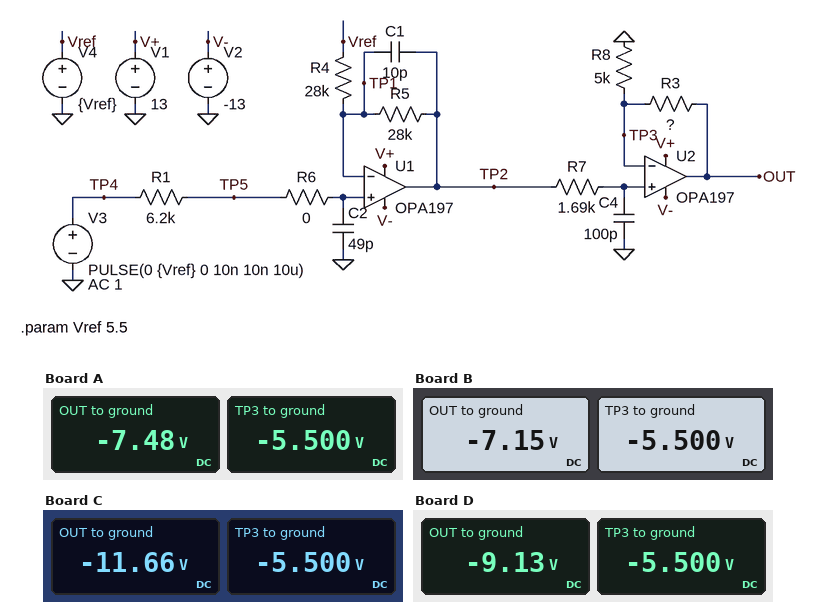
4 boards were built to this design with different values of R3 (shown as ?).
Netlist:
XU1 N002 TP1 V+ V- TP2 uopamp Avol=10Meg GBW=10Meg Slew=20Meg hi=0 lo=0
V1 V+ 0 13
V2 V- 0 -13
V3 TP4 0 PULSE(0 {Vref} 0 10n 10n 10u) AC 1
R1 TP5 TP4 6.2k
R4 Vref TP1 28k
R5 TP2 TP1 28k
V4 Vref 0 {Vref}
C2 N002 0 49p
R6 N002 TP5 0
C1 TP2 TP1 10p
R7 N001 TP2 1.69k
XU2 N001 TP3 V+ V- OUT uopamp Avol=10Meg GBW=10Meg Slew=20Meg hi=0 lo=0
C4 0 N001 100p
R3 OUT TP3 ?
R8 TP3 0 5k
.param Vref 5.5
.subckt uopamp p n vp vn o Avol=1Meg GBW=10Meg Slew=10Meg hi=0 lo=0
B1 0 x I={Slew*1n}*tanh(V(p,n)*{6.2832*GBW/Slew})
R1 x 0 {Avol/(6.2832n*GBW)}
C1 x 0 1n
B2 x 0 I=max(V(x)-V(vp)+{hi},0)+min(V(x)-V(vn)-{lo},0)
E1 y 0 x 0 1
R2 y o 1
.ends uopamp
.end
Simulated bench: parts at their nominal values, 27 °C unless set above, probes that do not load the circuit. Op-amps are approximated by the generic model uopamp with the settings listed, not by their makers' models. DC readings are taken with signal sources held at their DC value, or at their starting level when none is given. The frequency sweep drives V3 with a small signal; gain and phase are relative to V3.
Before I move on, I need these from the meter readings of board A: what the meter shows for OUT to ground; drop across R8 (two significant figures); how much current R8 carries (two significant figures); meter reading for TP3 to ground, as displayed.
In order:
-7.48 V
5.5 V
1.1 mA
-5.500 V
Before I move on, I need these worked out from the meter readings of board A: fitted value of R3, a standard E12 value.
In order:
1.8 kΩ
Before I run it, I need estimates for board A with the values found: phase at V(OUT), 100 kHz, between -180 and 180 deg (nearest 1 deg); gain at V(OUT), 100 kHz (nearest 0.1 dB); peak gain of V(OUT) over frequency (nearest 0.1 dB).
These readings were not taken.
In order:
-20 deg
4.9 dB
5.1 dB
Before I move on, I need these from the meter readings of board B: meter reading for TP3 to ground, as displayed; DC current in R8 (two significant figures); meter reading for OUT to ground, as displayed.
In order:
-5.500 V
1.1 mA
-7.15 V
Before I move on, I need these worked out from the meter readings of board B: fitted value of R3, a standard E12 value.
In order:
1.5 kΩ
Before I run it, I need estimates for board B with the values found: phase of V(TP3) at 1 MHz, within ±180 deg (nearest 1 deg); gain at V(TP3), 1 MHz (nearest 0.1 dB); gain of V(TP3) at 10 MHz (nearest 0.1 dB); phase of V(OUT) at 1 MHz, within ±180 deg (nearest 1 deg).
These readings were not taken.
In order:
-132 deg
-9.1 dB
-53.7 dB
-132 deg
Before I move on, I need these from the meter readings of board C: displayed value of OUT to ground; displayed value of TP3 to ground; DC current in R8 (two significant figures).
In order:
-11.66 V
-5.500 V
1.1 mA
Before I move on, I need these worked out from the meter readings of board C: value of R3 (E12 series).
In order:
5.6 kΩ
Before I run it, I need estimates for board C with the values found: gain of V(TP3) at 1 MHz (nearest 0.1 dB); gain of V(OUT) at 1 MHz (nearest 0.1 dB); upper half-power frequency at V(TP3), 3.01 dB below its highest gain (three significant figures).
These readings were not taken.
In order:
-9.2 dB
-2.7 dB
389 kHz
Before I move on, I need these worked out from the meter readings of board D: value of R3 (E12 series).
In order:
3.3 kΩ
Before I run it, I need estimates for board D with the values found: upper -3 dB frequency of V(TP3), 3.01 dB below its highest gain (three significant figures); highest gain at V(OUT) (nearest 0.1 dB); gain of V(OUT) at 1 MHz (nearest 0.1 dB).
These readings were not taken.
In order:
390 kHz
6.8 dB
-4.8 dB
